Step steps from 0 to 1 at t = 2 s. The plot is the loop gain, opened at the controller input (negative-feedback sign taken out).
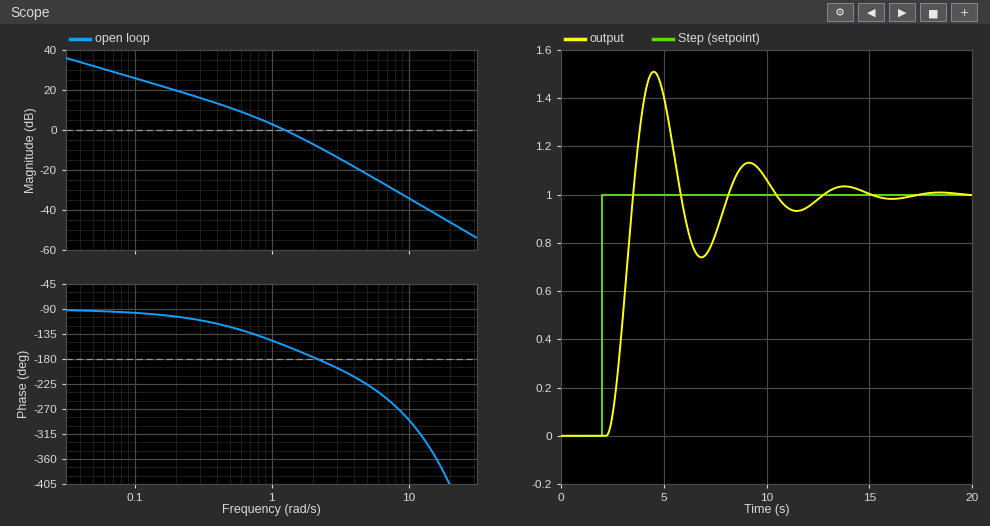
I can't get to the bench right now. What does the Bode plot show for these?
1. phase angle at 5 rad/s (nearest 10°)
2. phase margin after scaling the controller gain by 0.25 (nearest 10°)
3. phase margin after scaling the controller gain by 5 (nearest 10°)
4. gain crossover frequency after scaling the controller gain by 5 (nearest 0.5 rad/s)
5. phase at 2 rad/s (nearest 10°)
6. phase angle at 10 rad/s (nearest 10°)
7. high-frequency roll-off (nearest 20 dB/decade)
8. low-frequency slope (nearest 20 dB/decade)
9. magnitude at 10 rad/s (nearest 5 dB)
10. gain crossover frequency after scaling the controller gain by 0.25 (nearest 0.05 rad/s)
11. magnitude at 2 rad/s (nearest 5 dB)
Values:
-230°
60°
-20°
3.0 rad/s
-180°
-290°
-40 dB/decade
-20 dB/decade
-35 dB
0.45 rad/s
-5 dB
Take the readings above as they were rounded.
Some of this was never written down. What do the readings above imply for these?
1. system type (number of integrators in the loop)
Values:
1
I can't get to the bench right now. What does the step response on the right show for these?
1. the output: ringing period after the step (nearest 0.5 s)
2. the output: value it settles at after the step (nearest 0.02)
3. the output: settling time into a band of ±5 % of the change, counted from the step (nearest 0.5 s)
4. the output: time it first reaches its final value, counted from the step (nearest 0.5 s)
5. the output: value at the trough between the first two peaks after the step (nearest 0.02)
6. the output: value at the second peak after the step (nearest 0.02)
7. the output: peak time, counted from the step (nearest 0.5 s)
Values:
4.5 s
1.00
10.0 s
1.5 s
0.74
1.14
2.5 s
